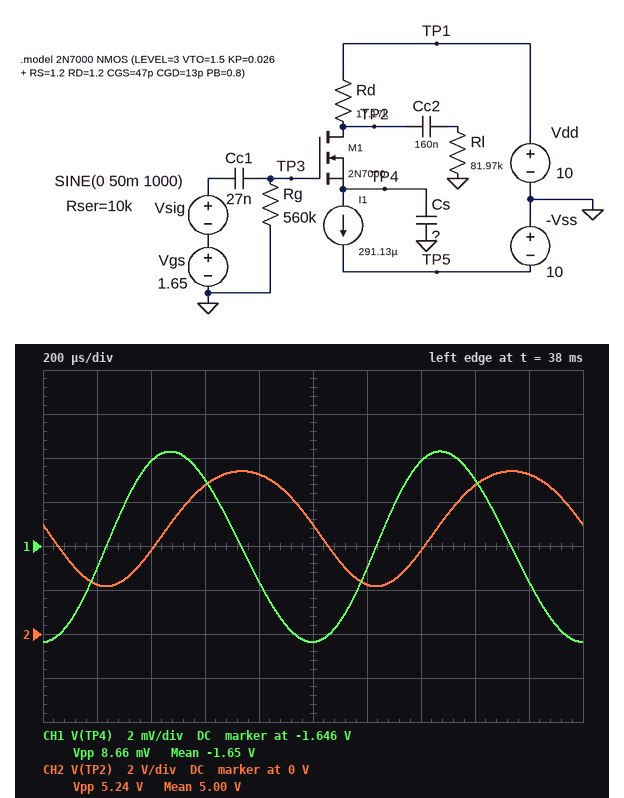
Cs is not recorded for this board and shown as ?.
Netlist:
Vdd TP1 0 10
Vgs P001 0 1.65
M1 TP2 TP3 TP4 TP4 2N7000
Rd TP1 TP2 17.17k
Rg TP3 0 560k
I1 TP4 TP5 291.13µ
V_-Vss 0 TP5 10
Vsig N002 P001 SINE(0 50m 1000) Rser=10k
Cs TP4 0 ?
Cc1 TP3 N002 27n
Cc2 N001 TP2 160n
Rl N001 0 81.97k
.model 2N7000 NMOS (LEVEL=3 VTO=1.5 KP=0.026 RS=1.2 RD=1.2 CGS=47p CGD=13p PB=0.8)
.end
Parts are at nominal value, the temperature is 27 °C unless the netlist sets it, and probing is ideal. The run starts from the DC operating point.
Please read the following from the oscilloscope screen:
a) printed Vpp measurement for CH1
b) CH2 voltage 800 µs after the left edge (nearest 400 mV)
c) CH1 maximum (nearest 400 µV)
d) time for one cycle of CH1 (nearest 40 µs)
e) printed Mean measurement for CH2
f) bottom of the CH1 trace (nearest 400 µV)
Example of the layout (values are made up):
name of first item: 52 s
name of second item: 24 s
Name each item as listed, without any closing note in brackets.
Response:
printed Vpp measurement for CH1: 8.66 mV
CH2 voltage 800 µs after the left edge: 7.2 V
CH1 maximum: -1.6416 V
time for one cycle of CH1: 1.00 ms
printed Mean measurement for CH2: 5.00 V
bottom of the CH1 trace: -1.6504 V
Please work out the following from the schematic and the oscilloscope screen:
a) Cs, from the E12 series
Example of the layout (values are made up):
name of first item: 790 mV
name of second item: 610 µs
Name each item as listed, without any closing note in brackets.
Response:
Cs, from the E12 series: 6.8 µF
